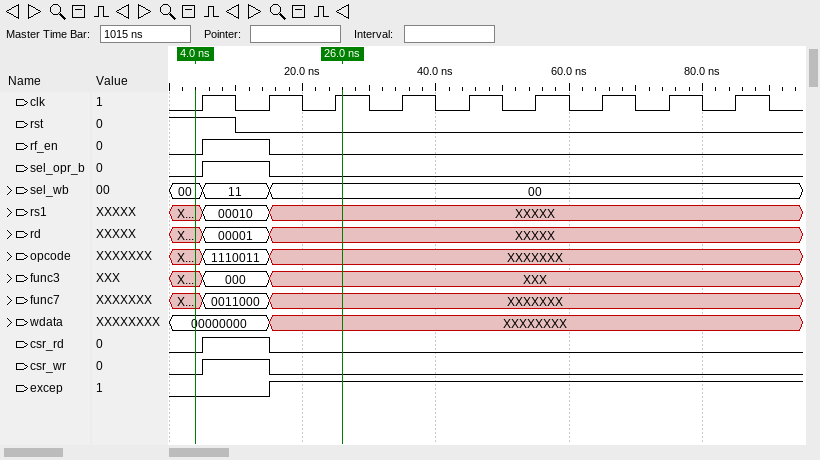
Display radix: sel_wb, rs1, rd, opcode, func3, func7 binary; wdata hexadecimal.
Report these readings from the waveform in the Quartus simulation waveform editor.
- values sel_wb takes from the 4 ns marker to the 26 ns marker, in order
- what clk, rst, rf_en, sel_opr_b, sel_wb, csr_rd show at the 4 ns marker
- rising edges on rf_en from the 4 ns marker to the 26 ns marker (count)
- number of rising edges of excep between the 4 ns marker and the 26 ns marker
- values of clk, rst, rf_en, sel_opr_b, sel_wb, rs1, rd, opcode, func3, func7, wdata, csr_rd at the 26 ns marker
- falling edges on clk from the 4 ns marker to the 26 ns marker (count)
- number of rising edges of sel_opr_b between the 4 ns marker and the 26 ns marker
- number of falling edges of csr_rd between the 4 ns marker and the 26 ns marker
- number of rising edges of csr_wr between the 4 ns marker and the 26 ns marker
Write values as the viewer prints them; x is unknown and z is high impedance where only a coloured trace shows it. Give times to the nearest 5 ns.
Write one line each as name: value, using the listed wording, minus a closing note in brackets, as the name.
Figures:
values sel_wb takes from the 4 ns marker to the 26 ns marker, in order: 00, 11, 00
what clk, rst, rf_en, sel_opr_b, sel_wb, csr_rd show at the 4 ns marker: clk=0, rst=1, rf_en=0, sel_opr_b=0, sel_wb=00, csr_rd=0
rising edges on rf_en from the 4 ns marker to the 26 ns marker: 1
number of rising edges of excep between the 4 ns marker and the 26 ns marker: 1
values of clk, rst, rf_en, sel_opr_b, sel_wb, rs1, rd, opcode, func3, func7, wdata, csr_rd at the 26 ns marker: clk=1, rst=0, rf_en=0, sel_opr_b=0, sel_wb=00, rs1=XXXXX, rd=XXXXX, opcode=XXXXXXX, func3=XXX, func7=XXXXXXX, wdata=XXXXXXXX, csr_rd=0
falling edges on clk from the 4 ns marker to the 26 ns marker: 2
number of rising edges of sel_opr_b between the 4 ns marker and the 26 ns marker: 1
number of falling edges of csr_rd between the 4 ns marker and the 26 ns marker: 1
number of rising edges of csr_wr between the 4 ns marker and the 26 ns marker: 1
